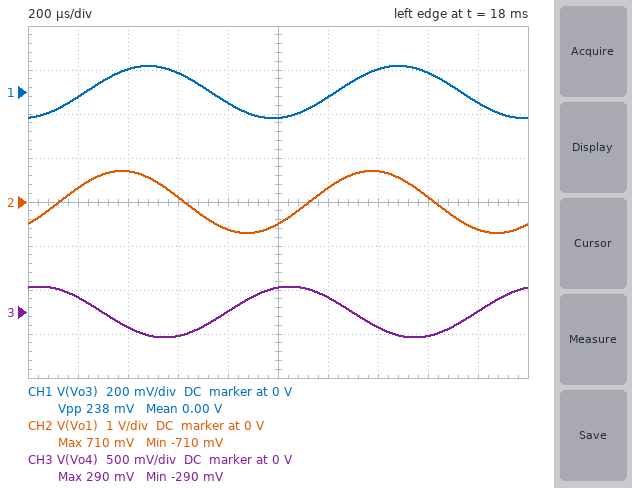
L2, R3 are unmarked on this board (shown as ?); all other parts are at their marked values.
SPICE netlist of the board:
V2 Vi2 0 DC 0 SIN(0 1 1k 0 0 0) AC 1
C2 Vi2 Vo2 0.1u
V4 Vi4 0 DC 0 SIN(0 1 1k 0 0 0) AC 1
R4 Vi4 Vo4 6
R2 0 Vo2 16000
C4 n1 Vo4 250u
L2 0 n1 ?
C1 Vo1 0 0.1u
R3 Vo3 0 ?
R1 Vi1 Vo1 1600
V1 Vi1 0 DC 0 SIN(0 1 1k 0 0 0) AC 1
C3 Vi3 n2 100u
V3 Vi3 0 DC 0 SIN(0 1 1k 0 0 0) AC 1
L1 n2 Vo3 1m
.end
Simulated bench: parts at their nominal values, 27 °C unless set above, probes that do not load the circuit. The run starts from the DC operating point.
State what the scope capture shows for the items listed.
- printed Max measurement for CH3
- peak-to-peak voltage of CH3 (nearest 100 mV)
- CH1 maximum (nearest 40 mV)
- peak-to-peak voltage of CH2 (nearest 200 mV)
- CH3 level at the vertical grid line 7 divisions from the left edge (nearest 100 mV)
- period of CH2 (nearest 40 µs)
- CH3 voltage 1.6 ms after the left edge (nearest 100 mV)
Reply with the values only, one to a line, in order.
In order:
290 mV
600 mV
120 mV
1.4 V
-200 mV
1.00 ms
-300 mV
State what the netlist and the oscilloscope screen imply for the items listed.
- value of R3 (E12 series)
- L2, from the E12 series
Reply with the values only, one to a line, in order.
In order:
0.56 Ω
390 µH
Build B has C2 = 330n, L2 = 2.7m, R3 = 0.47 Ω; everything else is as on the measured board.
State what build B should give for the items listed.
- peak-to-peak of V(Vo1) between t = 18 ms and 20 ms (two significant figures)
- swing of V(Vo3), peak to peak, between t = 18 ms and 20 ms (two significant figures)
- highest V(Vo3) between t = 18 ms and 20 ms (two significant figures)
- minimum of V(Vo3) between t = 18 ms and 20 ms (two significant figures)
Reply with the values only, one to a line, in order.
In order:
1.4 V
200 mV
100 mV
-100 mV
